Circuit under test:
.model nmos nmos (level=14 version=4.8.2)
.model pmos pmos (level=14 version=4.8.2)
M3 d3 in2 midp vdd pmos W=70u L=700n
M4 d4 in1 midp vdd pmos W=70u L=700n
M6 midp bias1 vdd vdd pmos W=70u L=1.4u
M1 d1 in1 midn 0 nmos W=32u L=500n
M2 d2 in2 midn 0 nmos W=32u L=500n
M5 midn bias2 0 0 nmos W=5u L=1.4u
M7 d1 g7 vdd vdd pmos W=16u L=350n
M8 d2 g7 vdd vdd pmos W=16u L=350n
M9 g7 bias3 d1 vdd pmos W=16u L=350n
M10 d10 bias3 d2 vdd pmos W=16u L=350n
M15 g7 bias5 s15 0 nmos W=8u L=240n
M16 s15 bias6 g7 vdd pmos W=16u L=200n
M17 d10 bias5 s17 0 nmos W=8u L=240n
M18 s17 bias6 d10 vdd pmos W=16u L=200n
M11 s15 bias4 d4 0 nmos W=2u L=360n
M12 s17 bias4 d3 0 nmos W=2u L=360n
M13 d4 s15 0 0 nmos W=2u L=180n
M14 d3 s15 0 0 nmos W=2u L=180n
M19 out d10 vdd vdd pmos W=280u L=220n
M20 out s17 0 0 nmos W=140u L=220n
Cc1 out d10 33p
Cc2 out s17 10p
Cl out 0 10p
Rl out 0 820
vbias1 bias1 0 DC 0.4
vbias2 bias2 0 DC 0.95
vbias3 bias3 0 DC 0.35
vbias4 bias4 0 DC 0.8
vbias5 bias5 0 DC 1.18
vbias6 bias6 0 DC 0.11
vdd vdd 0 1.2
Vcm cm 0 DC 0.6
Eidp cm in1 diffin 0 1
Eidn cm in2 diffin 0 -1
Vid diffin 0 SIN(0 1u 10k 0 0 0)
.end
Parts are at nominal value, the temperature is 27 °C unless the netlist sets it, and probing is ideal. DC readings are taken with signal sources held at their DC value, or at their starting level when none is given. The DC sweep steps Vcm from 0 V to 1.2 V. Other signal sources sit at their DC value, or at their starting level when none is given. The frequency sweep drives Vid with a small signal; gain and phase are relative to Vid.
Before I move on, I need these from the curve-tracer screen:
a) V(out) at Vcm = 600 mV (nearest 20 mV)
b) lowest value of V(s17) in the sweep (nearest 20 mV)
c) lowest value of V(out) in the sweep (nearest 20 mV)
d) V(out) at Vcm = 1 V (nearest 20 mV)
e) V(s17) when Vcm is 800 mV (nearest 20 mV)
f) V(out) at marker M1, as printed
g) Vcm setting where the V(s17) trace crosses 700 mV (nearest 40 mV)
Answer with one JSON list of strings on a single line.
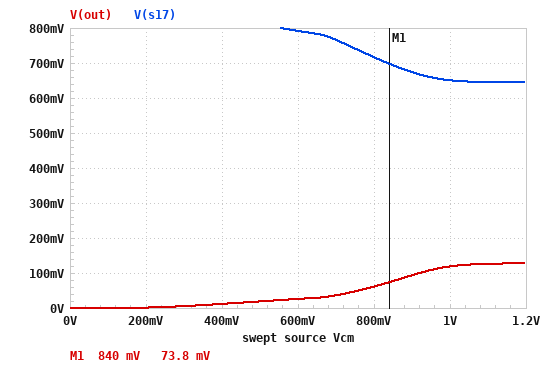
["20 mV", "640 mV", "0 V", "120 mV", "720 mV", "73.8 mV", "840 mV"]
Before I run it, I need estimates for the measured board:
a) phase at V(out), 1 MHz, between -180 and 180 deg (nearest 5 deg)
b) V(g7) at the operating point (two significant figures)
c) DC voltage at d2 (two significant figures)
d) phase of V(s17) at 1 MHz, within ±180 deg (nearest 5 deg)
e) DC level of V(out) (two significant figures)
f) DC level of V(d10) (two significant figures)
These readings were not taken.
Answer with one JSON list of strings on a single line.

["-80 deg", "790 mV", "790 mV", "100 deg", "26 mV", "790 mV"]
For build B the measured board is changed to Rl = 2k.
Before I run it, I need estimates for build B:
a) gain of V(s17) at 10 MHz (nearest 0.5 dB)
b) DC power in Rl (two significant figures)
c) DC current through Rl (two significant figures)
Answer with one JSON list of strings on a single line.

["2.0 dB", "340 nW", "13 µA"]
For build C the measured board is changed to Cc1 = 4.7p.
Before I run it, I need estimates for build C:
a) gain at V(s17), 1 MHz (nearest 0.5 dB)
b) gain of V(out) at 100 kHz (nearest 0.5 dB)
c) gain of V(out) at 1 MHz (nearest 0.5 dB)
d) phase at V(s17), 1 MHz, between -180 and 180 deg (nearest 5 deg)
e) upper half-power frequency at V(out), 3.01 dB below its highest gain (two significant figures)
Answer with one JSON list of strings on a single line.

["29.5 dB", "28.0 dB", "21.5 dB", "115 deg", "520 kHz"]
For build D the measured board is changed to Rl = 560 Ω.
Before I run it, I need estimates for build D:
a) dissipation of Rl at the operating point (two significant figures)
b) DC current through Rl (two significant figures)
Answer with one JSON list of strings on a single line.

["1.2 µW", "46 µA"]
